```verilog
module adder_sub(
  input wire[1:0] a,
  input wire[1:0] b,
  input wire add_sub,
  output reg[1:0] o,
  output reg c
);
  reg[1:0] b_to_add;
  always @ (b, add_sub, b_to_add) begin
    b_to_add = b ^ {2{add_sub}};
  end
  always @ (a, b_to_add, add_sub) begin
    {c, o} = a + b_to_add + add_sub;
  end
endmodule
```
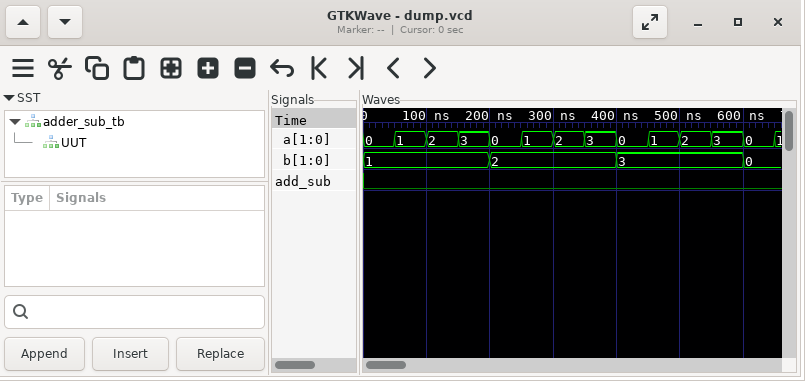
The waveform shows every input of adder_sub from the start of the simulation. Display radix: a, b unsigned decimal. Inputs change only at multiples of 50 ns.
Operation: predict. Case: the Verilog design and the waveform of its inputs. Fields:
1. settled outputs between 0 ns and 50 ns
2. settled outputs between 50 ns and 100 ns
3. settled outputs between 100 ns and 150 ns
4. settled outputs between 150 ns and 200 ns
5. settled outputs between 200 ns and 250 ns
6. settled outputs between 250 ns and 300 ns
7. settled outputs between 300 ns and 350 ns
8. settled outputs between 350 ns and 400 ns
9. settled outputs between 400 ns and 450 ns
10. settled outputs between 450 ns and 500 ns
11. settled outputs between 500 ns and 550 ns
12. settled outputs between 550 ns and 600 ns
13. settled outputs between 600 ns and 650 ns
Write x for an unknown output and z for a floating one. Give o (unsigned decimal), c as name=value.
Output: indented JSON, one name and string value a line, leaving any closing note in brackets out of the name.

{
  "settled outputs between 0 ns and 50 ns": "o=1, c=0",
  "settled outputs between 50 ns and 100 ns": "o=2, c=0",
  "settled outputs between 100 ns and 150 ns": "o=3, c=0",
  "settled outputs between 150 ns and 200 ns": "o=0, c=1",
  "settled outputs between 200 ns and 250 ns": "o=2, c=0",
  "settled outputs between 250 ns and 300 ns": "o=3, c=0",
  "settled outputs between 300 ns and 350 ns": "o=0, c=1",
  "settled outputs between 350 ns and 400 ns": "o=1, c=1",
  "settled outputs between 400 ns and 450 ns": "o=3, c=0",
  "settled outputs between 450 ns and 500 ns": "o=0, c=1",
  "settled outputs between 500 ns and 550 ns": "o=1, c=1",
  "settled outputs between 550 ns and 600 ns": "o=2, c=1",
  "settled outputs between 600 ns and 650 ns": "o=0, c=0"
}
